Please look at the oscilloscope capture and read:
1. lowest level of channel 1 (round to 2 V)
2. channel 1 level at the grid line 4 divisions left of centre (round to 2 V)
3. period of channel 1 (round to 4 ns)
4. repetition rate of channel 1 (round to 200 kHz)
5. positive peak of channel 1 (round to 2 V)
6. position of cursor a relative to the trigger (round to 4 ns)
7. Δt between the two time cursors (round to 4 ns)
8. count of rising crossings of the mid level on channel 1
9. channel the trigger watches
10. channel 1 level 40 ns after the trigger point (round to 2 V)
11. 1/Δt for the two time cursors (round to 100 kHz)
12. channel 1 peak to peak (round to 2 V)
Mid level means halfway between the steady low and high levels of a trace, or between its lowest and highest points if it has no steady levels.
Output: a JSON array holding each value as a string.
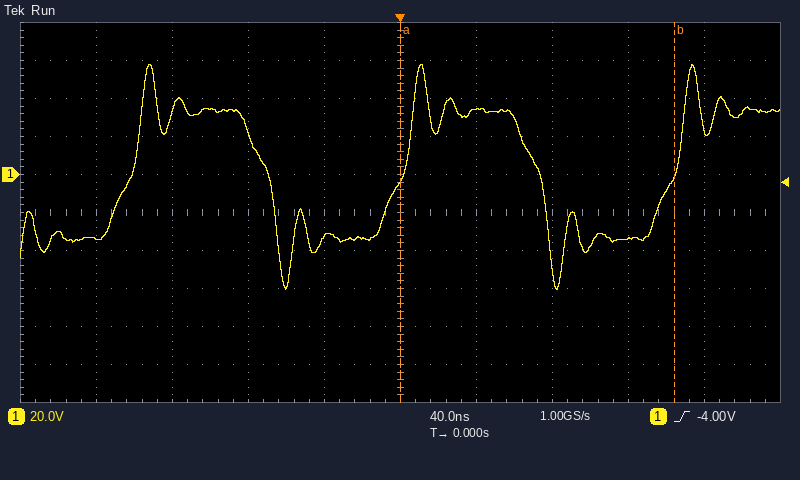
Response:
["-60 V", "-34 V", "144 ns", "7.0 MHz", "58 V", "0 ns", "144 ns", "3", "channel 1", "34 V", "6.9 MHz", "118 V"]
